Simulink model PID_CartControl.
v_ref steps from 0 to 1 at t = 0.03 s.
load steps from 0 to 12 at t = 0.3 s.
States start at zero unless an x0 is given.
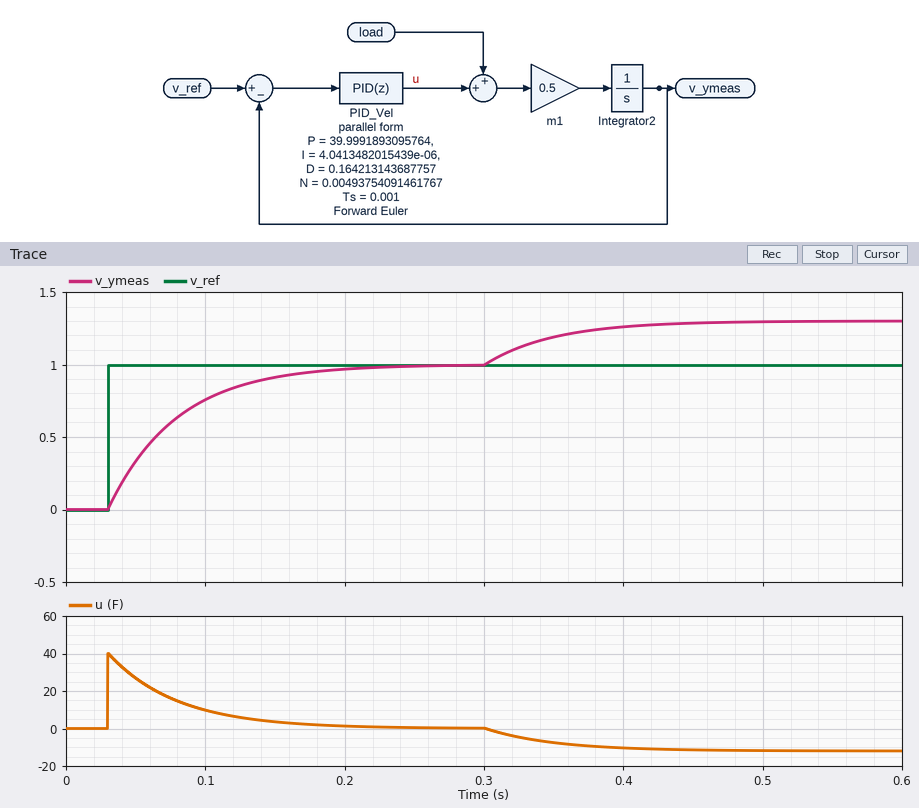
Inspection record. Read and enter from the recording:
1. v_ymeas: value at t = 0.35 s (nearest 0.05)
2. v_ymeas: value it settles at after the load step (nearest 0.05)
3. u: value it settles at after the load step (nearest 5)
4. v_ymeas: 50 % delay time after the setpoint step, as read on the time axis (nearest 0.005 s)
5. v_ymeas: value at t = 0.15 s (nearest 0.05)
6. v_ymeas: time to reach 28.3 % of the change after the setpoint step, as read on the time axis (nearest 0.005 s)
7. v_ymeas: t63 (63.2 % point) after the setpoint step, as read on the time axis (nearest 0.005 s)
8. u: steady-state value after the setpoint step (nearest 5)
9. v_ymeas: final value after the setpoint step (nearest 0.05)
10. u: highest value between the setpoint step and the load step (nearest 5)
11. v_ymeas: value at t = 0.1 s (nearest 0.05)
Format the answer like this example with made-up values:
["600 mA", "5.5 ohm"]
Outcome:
["1.20", "1.30", "-10", "0.065 s", "0.90", "0.045 s", "0.080 s", "0", "1.00", "40", "0.75"]
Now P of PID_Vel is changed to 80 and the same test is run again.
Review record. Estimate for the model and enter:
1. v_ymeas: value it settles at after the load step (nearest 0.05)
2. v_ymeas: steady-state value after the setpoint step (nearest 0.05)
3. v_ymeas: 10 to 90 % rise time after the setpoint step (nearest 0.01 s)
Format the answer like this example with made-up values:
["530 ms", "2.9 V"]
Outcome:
["1.15", "1.00", "0.05 s"]
